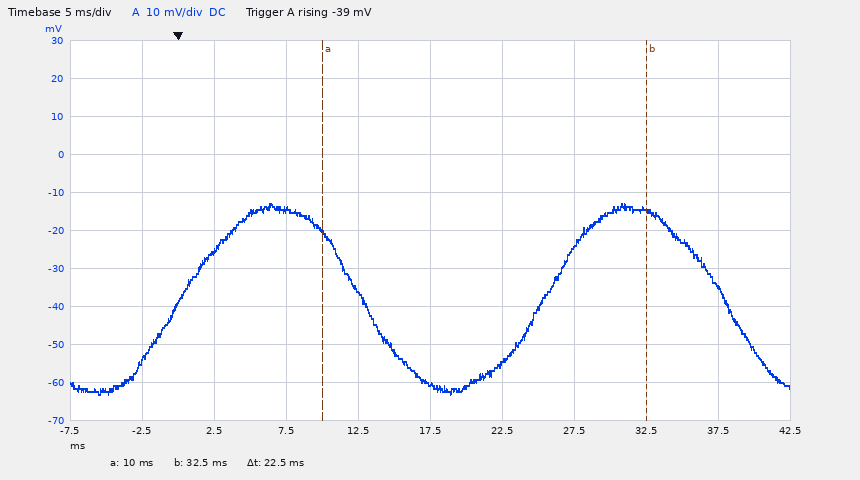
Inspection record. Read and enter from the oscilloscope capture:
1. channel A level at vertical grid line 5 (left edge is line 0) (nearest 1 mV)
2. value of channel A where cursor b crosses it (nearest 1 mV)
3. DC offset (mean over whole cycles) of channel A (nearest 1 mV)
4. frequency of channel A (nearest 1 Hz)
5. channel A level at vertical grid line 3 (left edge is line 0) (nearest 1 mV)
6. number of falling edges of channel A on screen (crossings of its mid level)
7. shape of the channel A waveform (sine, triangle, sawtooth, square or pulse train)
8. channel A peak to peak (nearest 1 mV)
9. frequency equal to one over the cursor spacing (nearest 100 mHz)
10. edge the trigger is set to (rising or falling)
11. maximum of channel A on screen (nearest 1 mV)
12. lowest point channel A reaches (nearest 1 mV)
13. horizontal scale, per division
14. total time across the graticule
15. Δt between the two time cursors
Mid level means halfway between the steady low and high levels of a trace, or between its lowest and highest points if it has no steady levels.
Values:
-60 mV
-15 mV
-38 mV
40 Hz
-14 mV
2
sine
50 mV
44.4 Hz
rising
-13 mV
-63 mV
5 ms
50 ms
22.5 ms
